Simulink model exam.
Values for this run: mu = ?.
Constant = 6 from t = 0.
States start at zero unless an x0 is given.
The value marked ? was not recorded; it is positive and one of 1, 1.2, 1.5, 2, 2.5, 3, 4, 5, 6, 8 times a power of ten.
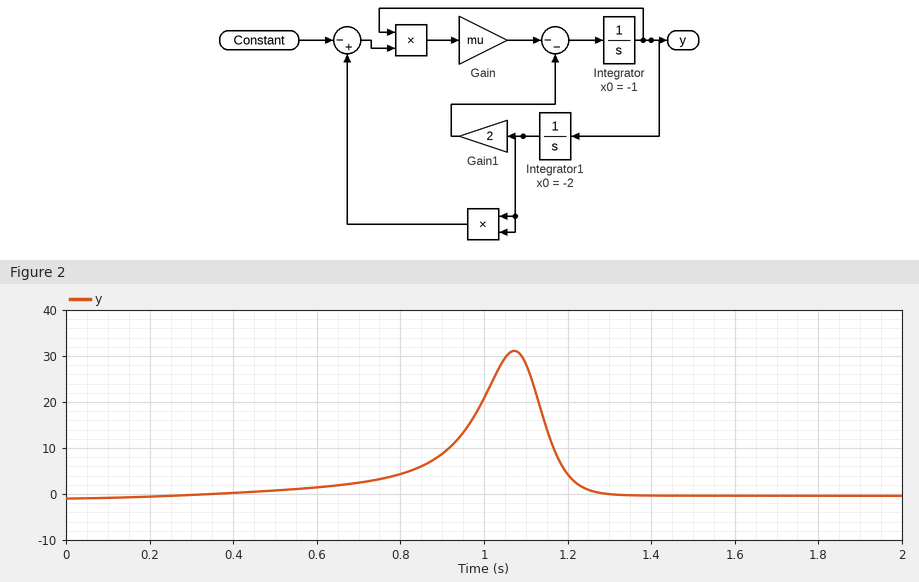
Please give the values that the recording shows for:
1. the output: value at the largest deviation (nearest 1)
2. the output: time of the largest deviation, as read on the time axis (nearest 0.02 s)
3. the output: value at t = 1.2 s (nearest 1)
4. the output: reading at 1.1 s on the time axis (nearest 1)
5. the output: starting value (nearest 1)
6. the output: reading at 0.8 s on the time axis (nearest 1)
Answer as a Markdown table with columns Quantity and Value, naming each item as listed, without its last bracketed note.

| Quantity | Value |
|---|---|
| the output: value at the largest deviation | 31 |
| the output: time of the largest deviation, as read on the time axis | 1.08 s |
| the output: value at t = 1.2 s | 4 |
| the output: reading at 1.1 s on the time axis | 28 |
| the output: starting value | -1 |
| the output: reading at 0.8 s on the time axis | 4 |
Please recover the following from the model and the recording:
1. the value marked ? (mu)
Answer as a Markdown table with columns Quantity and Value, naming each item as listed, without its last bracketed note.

| Quantity | Value |
|---|---|
| the value marked ? | 1.5 |
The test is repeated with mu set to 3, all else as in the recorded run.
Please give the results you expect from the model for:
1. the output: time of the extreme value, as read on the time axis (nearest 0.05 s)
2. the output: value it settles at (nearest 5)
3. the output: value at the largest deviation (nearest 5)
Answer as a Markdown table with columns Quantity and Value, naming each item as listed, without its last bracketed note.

| Quantity | Value |
|---|---|
| the output: time of the extreme value, as read on the time axis | 1.15 s |
| the output: value it settles at | 0 |
| the output: value at the largest deviation | 60 |
